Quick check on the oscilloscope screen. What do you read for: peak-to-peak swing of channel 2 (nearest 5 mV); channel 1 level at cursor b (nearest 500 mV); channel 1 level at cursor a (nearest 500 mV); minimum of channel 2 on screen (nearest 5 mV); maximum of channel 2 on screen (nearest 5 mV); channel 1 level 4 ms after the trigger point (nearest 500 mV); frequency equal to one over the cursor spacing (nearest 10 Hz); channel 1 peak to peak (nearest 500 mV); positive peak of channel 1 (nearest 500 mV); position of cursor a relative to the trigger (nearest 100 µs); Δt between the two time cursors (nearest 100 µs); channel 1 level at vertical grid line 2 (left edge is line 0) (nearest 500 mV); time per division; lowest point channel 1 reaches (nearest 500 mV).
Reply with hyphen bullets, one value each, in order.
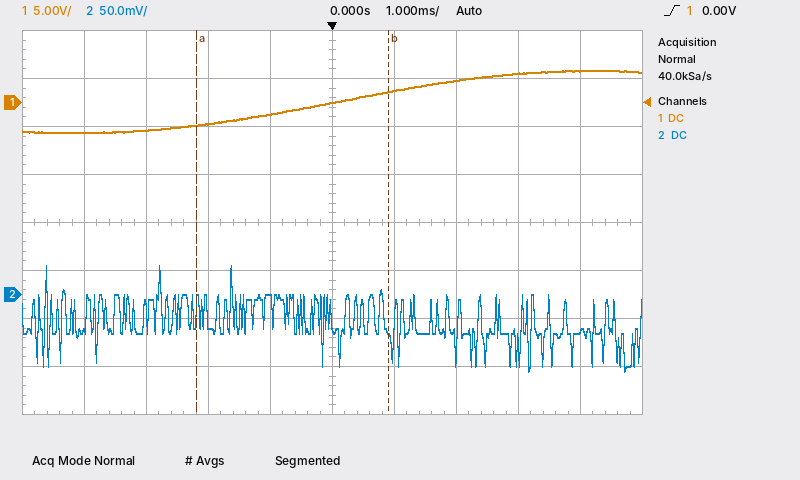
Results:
- 110 mV
- 1.0 V
- -2.5 V
- -80 mV
- 30 mV
- 3.5 V
- 320 Hz
- 6.5 V
- 3.5 V
- -2.2 ms
- 3.1 ms
- -3.0 V
- 1 ms
- -3.0 V
